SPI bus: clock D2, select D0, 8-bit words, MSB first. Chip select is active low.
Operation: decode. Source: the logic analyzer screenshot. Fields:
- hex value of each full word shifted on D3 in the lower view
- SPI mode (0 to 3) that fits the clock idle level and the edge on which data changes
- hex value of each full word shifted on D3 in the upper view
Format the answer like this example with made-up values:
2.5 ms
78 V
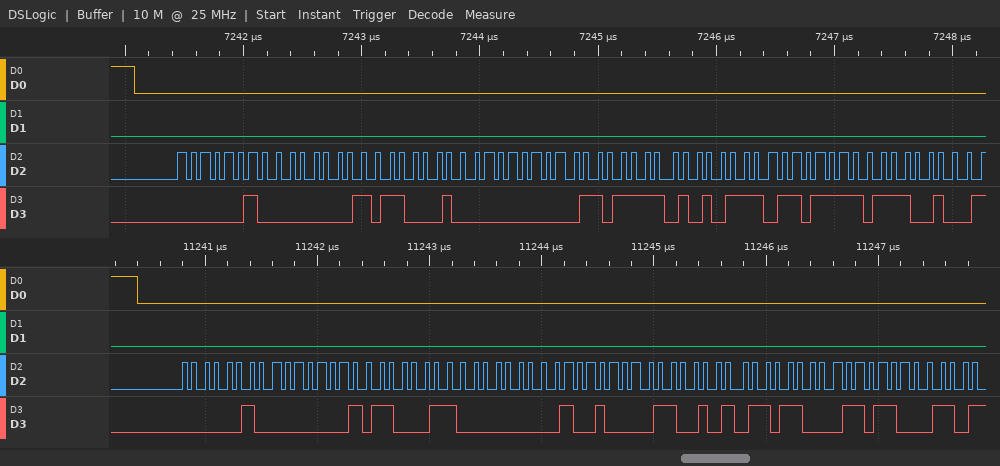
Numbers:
02, 01, 63, 00, 48, 65, 6C, 6C
0
02, 01, 62, 00, 6F, 57, 6F, 72
